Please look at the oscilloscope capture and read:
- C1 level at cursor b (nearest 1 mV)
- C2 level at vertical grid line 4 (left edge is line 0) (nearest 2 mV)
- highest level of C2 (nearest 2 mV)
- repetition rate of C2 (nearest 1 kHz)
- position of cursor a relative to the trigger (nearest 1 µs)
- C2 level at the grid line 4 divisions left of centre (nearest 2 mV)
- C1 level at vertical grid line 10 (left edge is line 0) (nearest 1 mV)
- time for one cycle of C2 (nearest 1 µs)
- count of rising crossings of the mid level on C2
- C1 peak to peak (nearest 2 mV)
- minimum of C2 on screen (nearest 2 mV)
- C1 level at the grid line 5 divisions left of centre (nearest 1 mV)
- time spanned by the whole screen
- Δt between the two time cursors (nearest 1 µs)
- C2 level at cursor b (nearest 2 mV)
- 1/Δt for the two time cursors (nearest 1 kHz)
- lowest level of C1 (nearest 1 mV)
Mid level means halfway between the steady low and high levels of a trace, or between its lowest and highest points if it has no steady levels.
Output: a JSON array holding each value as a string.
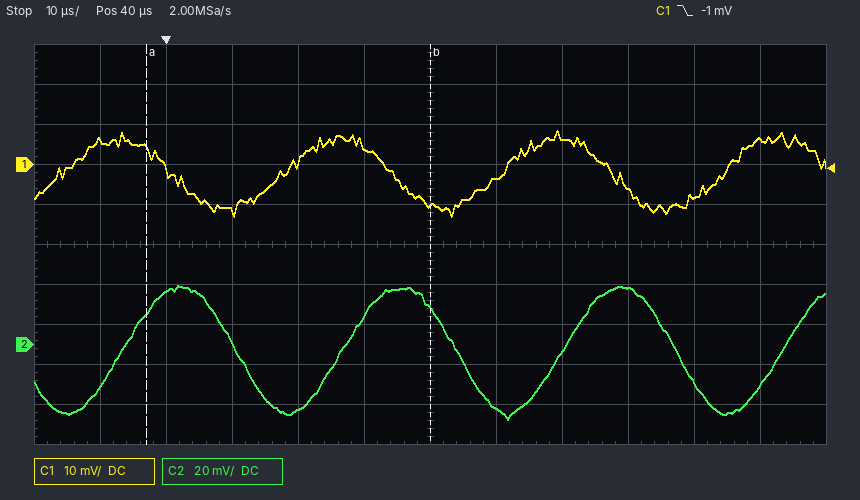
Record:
["-10 mV", "-32 mV", "30 mV", "30 kHz", "-3 µs", "26 mV", "-8 mV", "33 µs", "4", "22 mV", "-38 mV", "6 mV", "120 µs", "43 µs", "18 mV", "23 kHz", "-13 mV"]
